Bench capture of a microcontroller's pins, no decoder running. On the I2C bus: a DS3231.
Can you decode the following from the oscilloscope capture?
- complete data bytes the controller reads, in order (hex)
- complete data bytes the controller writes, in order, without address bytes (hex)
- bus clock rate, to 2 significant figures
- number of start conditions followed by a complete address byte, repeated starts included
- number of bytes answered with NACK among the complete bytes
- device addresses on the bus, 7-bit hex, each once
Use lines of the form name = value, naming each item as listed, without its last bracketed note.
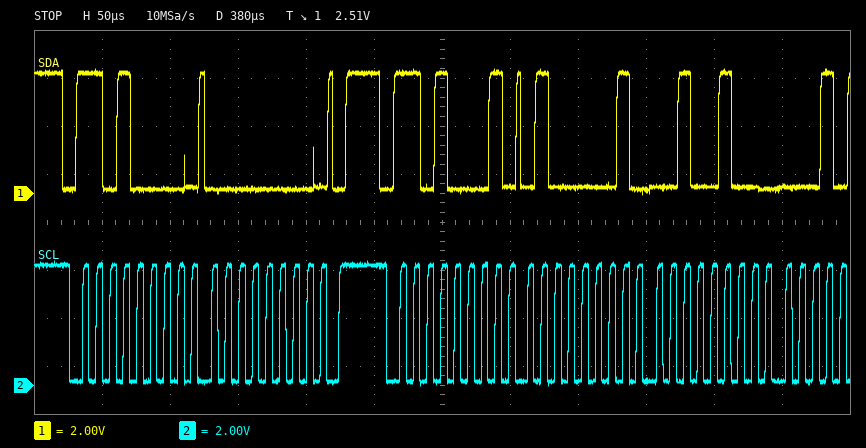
complete data bytes the controller reads, in order = 41 24
complete data bytes the controller writes, in order, without address bytes = 00
bus clock rate, to 2 significant figures = 100 kHz
number of start conditions followed by a complete address byte, repeated starts included = 2
number of bytes answered with NACK among the complete bytes = 0
device addresses on the bus, 7-bit hex, each once = 0x68
